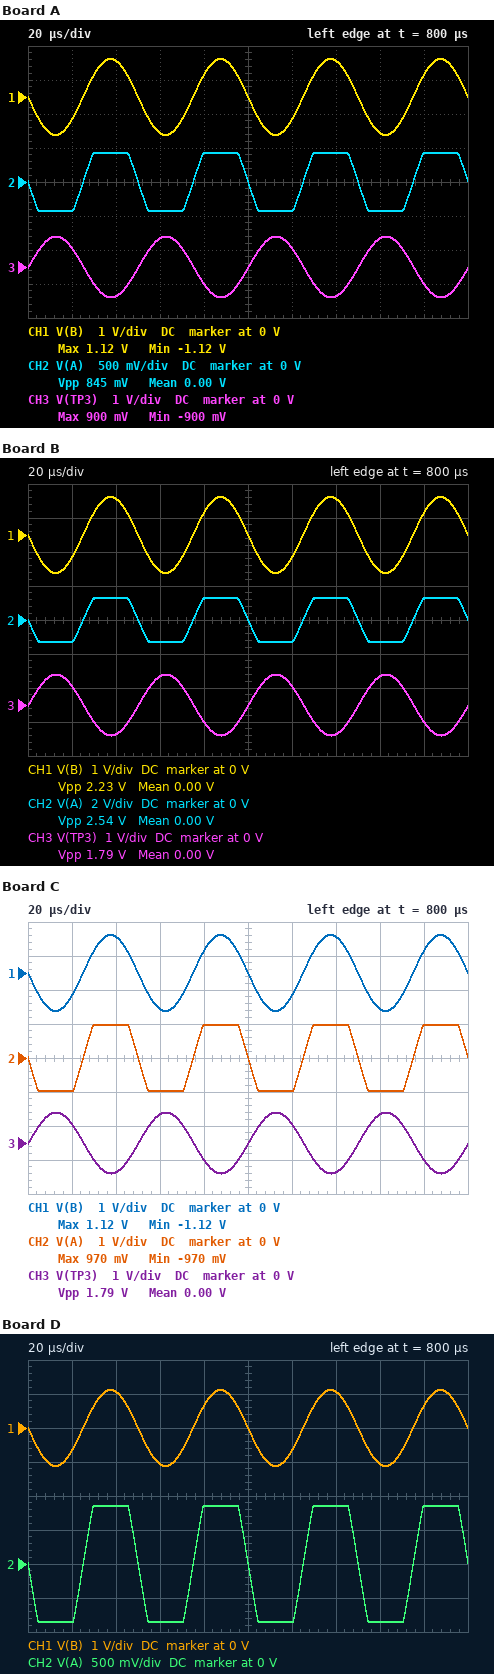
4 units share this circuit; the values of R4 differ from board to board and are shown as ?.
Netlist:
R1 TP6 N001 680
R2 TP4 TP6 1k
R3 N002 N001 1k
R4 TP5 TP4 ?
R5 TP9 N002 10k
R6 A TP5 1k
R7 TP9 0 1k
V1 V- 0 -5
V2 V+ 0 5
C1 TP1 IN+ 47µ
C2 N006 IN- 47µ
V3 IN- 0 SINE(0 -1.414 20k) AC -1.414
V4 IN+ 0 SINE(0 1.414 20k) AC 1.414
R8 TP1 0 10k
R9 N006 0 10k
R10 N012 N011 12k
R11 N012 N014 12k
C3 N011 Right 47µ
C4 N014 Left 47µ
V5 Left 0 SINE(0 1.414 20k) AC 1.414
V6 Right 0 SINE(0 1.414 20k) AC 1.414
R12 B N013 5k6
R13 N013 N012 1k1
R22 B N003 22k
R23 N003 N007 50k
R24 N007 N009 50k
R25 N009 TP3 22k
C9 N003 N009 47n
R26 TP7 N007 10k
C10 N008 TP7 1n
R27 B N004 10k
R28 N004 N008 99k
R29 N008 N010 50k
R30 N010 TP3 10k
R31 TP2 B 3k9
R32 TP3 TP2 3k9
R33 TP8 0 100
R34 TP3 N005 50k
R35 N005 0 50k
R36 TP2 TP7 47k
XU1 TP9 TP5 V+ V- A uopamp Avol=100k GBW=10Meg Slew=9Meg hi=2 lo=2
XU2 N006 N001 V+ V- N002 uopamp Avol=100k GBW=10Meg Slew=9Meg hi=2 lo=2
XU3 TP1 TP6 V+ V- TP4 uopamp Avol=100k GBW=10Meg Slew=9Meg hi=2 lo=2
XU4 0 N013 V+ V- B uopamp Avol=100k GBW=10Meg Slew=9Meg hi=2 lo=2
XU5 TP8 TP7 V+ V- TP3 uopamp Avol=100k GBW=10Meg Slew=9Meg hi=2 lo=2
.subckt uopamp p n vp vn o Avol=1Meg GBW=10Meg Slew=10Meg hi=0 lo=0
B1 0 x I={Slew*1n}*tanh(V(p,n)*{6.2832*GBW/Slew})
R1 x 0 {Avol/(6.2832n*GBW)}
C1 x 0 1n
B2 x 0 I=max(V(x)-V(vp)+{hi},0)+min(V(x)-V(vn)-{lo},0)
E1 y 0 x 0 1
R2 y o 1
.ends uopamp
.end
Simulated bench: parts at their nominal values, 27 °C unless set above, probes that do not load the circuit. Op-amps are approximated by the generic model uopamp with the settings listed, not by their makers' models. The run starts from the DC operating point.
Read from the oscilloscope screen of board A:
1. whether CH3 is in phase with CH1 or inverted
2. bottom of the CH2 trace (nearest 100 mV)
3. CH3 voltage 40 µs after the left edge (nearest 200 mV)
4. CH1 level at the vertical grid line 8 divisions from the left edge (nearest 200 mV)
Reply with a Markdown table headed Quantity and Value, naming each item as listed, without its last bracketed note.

| Quantity | Value |
|---|---|
| whether CH3 is in phase with CH1 or inverted | inverted |
| bottom of the CH2 trace | -400 mV |
| CH3 voltage 40 µs after the left edge | -800 mV |
| CH1 level at the vertical grid line 8 divisions from the left edge | -1.0 V |
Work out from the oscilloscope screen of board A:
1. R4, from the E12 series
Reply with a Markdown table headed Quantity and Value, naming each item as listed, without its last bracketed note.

| Quantity | Value |
|---|---|
| R4, from the E12 series | 22 kΩ |
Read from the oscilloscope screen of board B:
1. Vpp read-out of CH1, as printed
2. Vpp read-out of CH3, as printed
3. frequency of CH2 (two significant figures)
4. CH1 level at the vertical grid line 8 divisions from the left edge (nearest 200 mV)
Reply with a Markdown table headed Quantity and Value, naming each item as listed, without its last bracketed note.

| Quantity | Value |
|---|---|
| Vpp read-out of CH1, as printed | 2.23 V |
| Vpp read-out of CH3, as printed | 1.79 V |
| frequency of CH2 | 20 kHz |
| CH1 level at the vertical grid line 8 divisions from the left edge | -1.0 V |
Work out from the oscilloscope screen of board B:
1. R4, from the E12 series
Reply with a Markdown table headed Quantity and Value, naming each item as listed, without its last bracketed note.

| Quantity | Value |
|---|---|
| R4, from the E12 series | 3.3 kΩ |
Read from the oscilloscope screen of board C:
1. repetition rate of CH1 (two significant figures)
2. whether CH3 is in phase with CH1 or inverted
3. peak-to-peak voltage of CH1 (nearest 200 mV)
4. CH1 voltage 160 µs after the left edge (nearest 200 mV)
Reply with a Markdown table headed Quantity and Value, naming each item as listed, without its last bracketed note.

| Quantity | Value |
|---|---|
| repetition rate of CH1 | 20 kHz |
| whether CH3 is in phase with CH1 or inverted | inverted |
| peak-to-peak voltage of CH1 | 2.2 V |
| CH1 voltage 160 µs after the left edge | -1.0 V |
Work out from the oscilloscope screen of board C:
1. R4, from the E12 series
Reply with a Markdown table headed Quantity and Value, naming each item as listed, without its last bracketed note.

| Quantity | Value |
|---|---|
| R4, from the E12 series | 4.7 kΩ |
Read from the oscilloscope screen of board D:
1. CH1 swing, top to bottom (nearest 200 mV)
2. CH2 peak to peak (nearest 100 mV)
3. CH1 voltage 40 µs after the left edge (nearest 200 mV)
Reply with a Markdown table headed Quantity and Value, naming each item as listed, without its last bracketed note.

| Quantity | Value |
|---|---|
| CH1 swing, top to bottom | 2.2 V |
| CH2 peak to peak | 1.7 V |
| CH1 voltage 40 µs after the left edge | 1.0 V |
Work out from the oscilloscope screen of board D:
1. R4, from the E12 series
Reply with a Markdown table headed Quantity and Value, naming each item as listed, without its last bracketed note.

| Quantity | Value |
|---|---|
| R4, from the E12 series | 5.6 kΩ |
